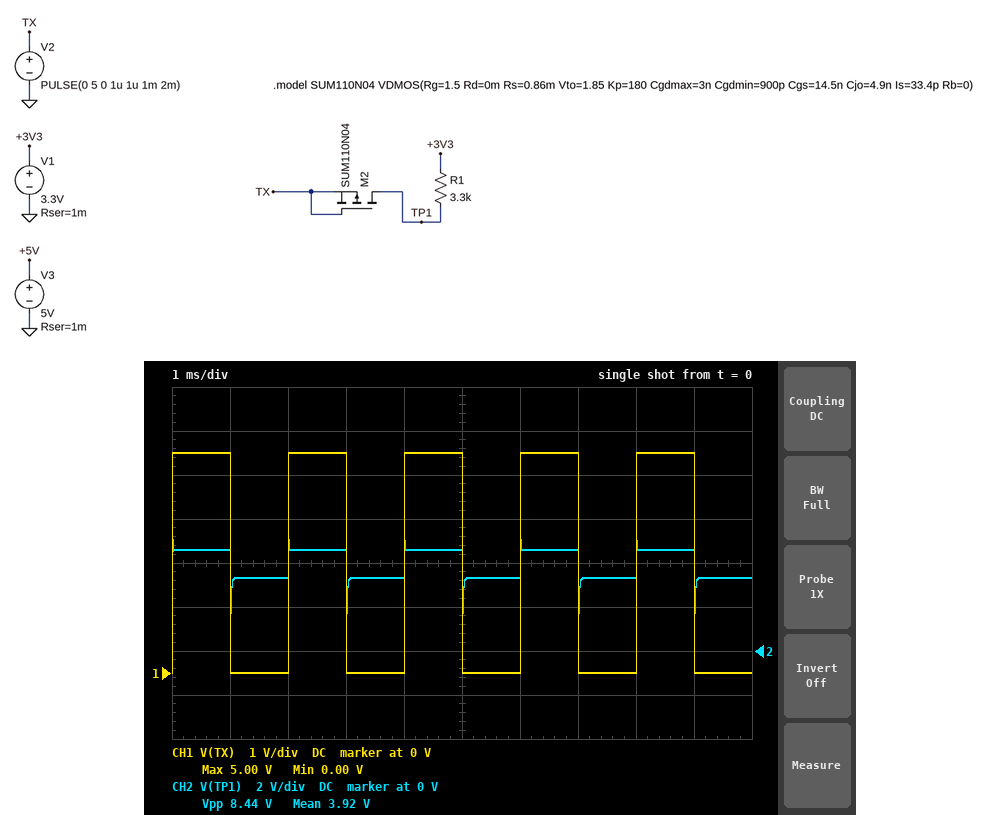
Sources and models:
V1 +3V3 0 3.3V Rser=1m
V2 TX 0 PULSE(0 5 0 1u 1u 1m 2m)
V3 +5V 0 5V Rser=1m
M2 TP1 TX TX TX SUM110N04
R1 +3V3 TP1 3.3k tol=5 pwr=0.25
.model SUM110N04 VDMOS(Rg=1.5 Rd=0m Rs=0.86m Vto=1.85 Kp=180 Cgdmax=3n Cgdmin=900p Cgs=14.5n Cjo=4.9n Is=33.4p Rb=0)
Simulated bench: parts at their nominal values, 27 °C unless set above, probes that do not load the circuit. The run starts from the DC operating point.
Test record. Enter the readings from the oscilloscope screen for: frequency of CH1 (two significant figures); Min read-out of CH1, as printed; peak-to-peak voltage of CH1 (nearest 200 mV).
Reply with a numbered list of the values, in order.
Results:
1. 500 Hz
2. 0.00 V
3. 5.0 V
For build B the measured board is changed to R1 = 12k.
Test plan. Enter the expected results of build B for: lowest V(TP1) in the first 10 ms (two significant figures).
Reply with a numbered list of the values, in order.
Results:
1. -370 mV
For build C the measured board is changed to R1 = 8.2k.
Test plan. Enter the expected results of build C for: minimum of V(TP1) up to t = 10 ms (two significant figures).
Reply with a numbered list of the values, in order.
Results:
1. -370 mV
